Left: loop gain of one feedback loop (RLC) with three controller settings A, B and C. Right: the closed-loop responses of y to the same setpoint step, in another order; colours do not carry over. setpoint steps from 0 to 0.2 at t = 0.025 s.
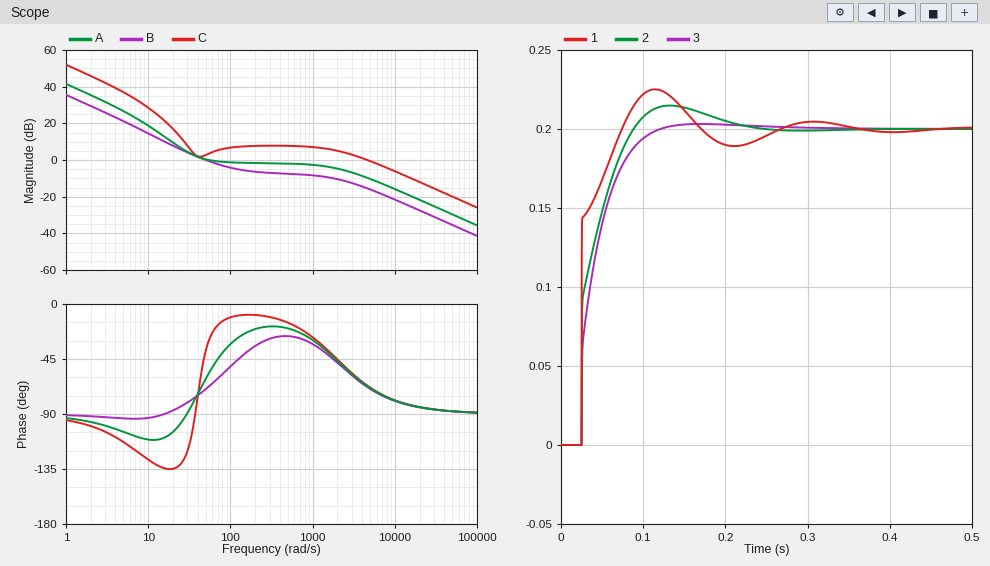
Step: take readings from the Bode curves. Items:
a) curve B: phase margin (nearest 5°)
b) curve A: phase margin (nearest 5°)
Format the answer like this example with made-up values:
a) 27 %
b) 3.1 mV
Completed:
a) 110°
b) 125°
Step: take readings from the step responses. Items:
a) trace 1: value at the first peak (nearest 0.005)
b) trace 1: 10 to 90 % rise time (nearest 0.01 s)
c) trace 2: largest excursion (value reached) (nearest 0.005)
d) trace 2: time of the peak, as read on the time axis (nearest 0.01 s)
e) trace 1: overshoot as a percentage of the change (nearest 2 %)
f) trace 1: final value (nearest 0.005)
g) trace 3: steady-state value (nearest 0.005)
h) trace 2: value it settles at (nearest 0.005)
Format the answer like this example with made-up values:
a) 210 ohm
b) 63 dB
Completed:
a) 0.225
b) 0.03 s
c) 0.215
d) 0.13 s
e) 12 %
f) 0.200
g) 0.200
h) 0.200
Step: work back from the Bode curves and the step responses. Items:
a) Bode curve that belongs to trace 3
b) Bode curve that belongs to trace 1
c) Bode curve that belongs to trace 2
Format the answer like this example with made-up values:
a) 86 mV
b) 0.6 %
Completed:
a) B
b) C
c) A
